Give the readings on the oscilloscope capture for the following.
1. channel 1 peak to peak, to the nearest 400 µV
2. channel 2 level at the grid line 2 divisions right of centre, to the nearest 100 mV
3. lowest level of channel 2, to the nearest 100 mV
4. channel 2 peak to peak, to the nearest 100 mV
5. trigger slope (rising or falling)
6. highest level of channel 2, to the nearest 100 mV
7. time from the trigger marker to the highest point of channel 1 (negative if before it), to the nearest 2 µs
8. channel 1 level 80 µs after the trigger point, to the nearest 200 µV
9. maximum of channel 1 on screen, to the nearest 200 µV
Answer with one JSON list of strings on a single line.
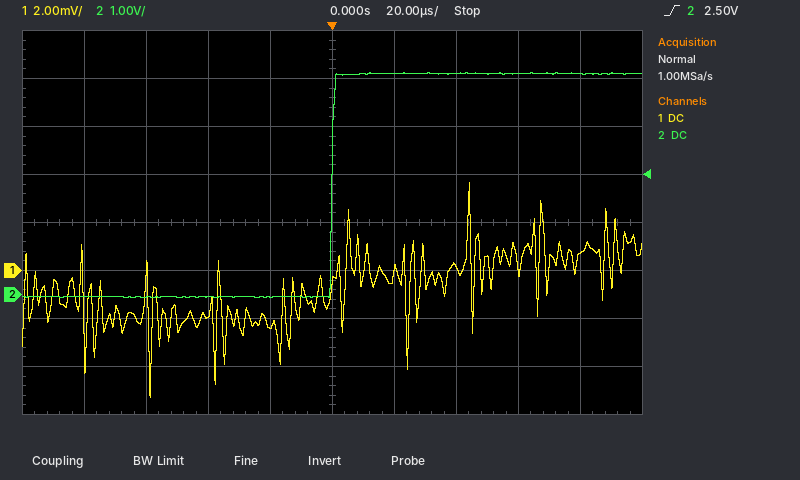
["8.8 mV", "4.6 V", "-100 mV", "4.7 V", "rising", "4.6 V", "+44 µs", "600 µV", "3.6 mV"]
